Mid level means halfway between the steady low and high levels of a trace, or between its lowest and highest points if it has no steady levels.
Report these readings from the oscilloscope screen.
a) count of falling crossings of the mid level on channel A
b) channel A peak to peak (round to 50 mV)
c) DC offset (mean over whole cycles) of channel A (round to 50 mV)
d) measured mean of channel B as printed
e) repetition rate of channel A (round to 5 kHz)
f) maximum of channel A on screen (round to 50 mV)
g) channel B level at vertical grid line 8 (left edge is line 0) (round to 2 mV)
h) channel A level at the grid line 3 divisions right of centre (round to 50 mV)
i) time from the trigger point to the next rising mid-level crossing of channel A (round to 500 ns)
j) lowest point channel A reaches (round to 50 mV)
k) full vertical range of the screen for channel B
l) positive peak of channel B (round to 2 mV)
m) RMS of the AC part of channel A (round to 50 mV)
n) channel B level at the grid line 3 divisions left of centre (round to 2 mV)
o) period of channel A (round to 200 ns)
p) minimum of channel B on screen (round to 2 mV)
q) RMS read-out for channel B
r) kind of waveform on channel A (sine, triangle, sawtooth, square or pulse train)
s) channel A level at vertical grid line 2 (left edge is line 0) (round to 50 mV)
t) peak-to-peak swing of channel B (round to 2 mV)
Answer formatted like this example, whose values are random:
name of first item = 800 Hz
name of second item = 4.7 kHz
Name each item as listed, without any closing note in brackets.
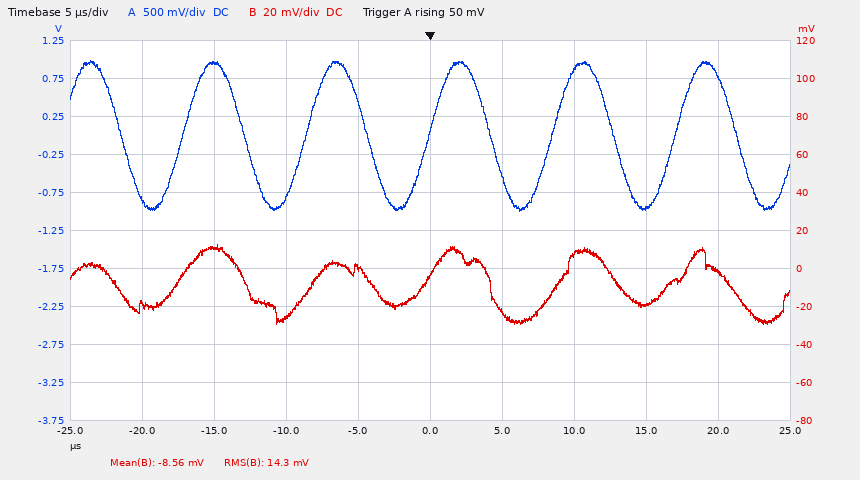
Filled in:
count of falling crossings of the mid level on channel A = 6
channel A peak to peak = 2.00 V
DC offset (mean over whole cycles) of channel A = 0 mV
measured mean of channel B as printed = -8.56 mV
repetition rate of channel A = 115 kHz
maximum of channel A on screen = 1.00 V
channel B level at vertical grid line 8 (left edge is line 0) = -20 mV
channel A level at the grid line 3 divisions right of centre = -950 mV
time from the trigger point to the next rising mid-level crossing of channel A = 8.5 µs
lowest point channel A reaches = -1.00 V
full vertical range of the screen for channel B = 200 mV
positive peak of channel B = 12 mV
RMS of the AC part of channel A = 700 mV
channel B level at the grid line 3 divisions left of centre = 10 mV
period of channel A = 8.6 µs
minimum of channel B on screen = -30 mV
RMS read-out for channel B = 14.3 mV
kind of waveform on channel A = sine
channel A level at vertical grid line 2 (left edge is line 0) = 950 mV
peak-to-peak swing of channel B = 42 mV
